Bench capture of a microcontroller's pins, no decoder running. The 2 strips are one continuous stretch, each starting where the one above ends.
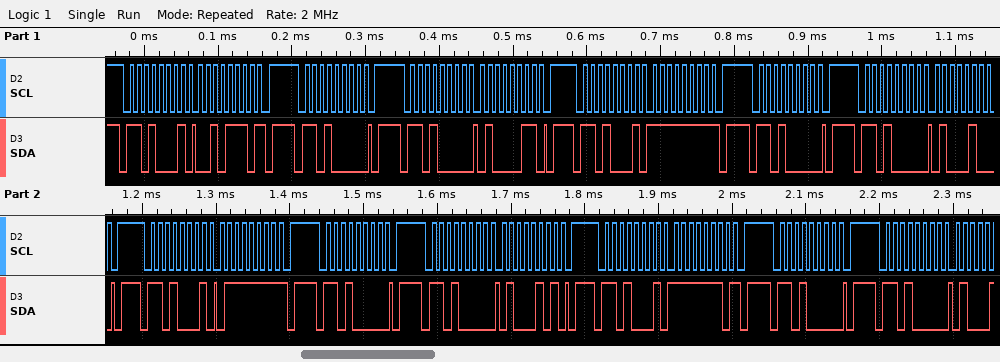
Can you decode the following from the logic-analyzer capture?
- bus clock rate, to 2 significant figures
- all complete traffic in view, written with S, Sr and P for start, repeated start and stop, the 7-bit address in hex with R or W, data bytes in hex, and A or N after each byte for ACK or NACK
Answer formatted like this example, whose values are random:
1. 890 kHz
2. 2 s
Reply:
1. 100 kHz
2. S 68R A 2E N P S 68W A P S 68W A 43 A P S 68R A FF N P S 68W A P S 68W A 44 A P S 68R A 7F N P S 68W A P S 68W A 45 A P S 68R A FE N P S 68W A P S 68W A
